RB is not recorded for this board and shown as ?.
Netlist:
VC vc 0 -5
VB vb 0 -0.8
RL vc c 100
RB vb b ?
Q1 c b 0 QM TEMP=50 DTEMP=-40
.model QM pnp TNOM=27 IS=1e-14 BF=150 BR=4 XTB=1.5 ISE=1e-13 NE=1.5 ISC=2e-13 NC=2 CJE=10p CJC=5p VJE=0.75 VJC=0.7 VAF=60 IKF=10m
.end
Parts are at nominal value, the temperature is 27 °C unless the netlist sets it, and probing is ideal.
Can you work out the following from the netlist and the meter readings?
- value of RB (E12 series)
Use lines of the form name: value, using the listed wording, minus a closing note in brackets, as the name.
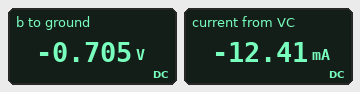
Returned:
value of RB: 560 Ω
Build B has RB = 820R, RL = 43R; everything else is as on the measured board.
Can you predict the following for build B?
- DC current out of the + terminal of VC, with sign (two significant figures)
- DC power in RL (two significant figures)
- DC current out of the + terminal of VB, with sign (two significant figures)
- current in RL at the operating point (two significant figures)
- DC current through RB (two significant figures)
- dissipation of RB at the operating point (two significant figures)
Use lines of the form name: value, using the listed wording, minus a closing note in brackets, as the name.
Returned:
DC current out of the + terminal of VC, with sign: -10 mA
DC power in RL: 4.5 mW
DC current out of the + terminal of VB, with sign: -130 µA
current in RL at the operating point: 10 mA
DC current through RB: 130 µA
dissipation of RB at the operating point: 13 µW
